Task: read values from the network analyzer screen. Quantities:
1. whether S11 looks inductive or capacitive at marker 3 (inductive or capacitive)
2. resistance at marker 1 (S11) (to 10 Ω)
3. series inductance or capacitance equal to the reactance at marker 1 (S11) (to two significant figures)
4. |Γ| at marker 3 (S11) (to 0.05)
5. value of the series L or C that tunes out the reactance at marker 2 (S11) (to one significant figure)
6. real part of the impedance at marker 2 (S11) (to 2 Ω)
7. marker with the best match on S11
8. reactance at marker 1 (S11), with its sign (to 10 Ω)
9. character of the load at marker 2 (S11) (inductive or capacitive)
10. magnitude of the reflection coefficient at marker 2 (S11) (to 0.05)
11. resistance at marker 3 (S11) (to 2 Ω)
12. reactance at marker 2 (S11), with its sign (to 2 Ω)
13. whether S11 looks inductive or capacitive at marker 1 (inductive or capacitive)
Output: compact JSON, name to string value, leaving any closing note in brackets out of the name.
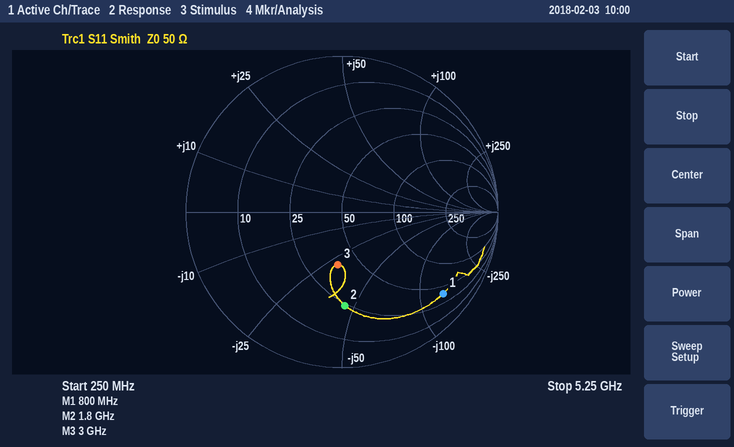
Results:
{"whether S11 looks inductive or capacitive at marker 3": "capacitive", "resistance at marker 1 (S11)": "40 Ω", "series inductance or capacitance equal to the reactance at marker 1 (S11)": "1.5 pF", "|Γ| at marker 3 (S11)": "0.35", "value of the series L or C that tunes out the reactance at marker 2 (S11)": "4 nH", "real part of the impedance at marker 2 (S11)": "24 Ω", "marker with the best match on S11": "marker 3", "reactance at marker 1 (S11), with its sign": "-130 Ω", "character of the load at marker 2 (S11)": "capacitive", "magnitude of the reflection coefficient at marker 2 (S11)": "0.60", "resistance at marker 3 (S11)": "38 Ω", "reactance at marker 2 (S11), with its sign": "-46 Ω", "whether S11 looks inductive or capacitive at marker 1": "capacitive"}
